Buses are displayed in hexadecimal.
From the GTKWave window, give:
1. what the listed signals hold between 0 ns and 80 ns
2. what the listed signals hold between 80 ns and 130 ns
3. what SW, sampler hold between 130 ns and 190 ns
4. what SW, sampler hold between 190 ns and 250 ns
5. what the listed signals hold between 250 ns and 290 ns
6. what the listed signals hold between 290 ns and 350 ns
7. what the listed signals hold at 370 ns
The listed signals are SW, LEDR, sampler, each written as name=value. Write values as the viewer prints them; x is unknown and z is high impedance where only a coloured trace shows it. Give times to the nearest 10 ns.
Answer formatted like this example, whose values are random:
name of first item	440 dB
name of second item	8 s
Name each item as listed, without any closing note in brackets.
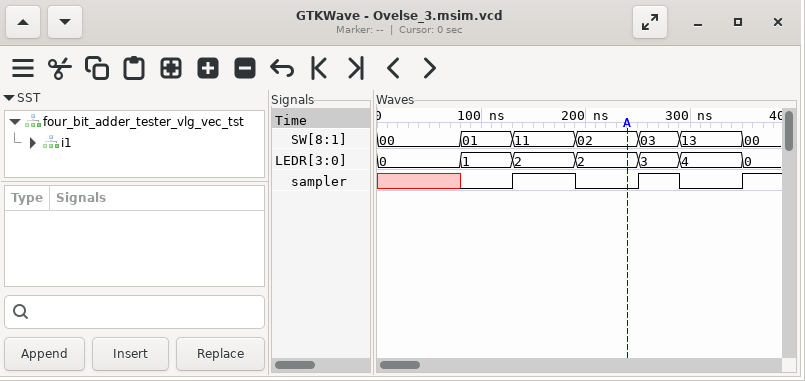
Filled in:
what the listed signals hold between 0 ns and 80 ns	SW=00, LEDR=0, sampler=x
what the listed signals hold between 80 ns and 130 ns	SW=01, LEDR=1, sampler=0
what SW, sampler hold between 130 ns and 190 ns	SW=11, sampler=1
what SW, sampler hold between 190 ns and 250 ns	SW=02, sampler=0
what the listed signals hold between 250 ns and 290 ns	SW=03, LEDR=3, sampler=1
what the listed signals hold between 290 ns and 350 ns	SW=13, LEDR=4, sampler=0
what the listed signals hold at 370 ns	SW=00, LEDR=0, sampler=1
